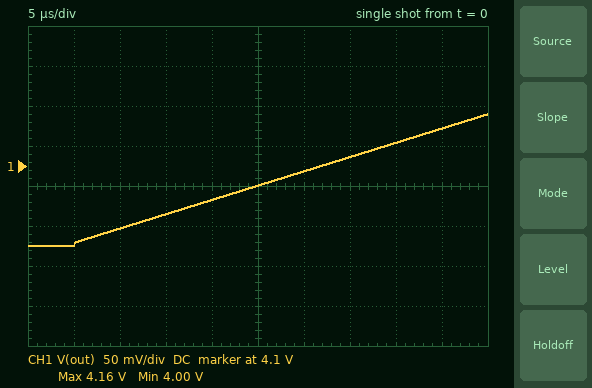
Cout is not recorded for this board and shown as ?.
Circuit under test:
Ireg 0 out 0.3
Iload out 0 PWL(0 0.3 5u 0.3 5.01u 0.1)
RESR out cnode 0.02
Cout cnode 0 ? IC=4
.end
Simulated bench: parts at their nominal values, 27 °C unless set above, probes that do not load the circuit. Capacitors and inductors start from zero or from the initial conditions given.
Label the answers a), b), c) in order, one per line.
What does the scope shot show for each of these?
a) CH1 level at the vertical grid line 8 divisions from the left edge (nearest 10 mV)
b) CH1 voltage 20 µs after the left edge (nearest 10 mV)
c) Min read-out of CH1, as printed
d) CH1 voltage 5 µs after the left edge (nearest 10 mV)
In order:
a) 4.13 V
b) 4.06 V
c) 4.00 V
d) 4.00 V
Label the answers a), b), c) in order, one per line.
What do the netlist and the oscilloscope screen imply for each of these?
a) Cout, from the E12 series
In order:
a) 56 µF
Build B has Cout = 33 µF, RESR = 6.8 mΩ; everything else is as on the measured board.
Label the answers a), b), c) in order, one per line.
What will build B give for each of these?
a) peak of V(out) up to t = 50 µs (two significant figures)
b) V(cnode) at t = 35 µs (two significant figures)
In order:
a) 4.3 V
b) 4.2 V
